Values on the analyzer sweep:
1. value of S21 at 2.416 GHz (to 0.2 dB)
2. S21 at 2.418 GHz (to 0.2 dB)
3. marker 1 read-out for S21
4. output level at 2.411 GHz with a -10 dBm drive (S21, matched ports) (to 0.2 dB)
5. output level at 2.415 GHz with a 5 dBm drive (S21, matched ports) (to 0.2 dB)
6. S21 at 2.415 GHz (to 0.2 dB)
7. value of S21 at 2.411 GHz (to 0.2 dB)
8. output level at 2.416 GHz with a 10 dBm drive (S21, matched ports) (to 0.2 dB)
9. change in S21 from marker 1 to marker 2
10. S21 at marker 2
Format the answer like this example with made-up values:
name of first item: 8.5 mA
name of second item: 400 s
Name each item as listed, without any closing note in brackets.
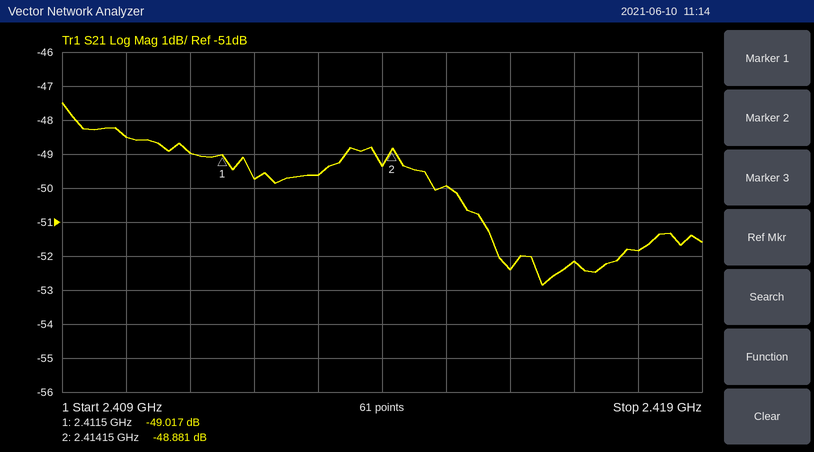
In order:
value of S21 at 2.416 GHz: -52.4 dB
S21 at 2.418 GHz: -51.8 dB
marker 1 read-out for S21: -49.017 dB
output level at 2.411 GHz with a -10 dBm drive (S21, matched ports): -59.0 dBm
output level at 2.415 GHz with a 5 dBm drive (S21, matched ports): -45.0 dBm
S21 at 2.415 GHz: -50.0 dB
value of S21 at 2.411 GHz: -49.0 dB
output level at 2.416 GHz with a 10 dBm drive (S21, matched ports): -42.4 dBm
change in S21 from marker 1 to marker 2: 0.136 dB
S21 at marker 2: -48.881 dB
